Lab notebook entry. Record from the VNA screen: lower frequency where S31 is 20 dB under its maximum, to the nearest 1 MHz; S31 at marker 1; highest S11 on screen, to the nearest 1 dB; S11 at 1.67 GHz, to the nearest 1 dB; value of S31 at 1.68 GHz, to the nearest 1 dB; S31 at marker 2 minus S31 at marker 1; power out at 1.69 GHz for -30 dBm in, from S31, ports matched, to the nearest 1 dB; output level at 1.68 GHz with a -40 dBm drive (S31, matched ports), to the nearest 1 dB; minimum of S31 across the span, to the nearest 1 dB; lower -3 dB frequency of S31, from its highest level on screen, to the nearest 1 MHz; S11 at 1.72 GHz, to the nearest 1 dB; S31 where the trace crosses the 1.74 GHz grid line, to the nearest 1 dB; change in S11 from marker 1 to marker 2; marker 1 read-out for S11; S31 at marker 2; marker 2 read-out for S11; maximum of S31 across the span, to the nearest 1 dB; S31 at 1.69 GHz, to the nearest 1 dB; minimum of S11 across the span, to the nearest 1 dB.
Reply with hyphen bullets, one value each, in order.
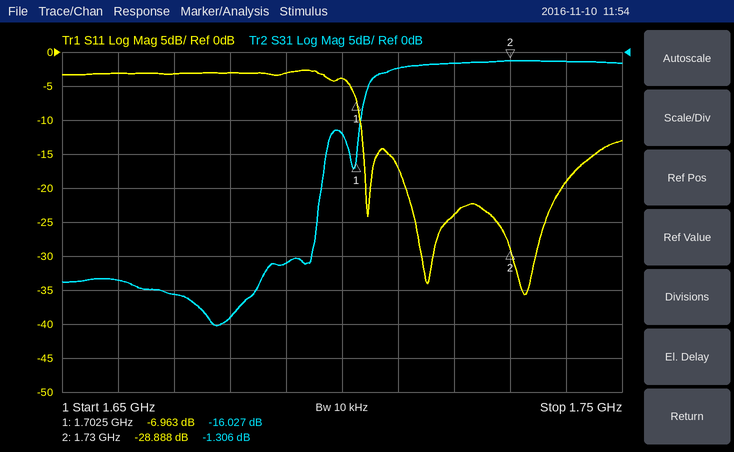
- 1.696 GHz
- -16.027 dB
- -3 dB
- -3 dB
- -39 dB
- 14.721 dB
- -61 dBm
- -79 dBm
- -40 dB
- 1.705 GHz
- -24 dB
- -1 dB
- -21.925 dB
- -6.963 dB
- -1.306 dB
- -28.888 dB
- -1 dB
- -31 dB
- -36 dB
